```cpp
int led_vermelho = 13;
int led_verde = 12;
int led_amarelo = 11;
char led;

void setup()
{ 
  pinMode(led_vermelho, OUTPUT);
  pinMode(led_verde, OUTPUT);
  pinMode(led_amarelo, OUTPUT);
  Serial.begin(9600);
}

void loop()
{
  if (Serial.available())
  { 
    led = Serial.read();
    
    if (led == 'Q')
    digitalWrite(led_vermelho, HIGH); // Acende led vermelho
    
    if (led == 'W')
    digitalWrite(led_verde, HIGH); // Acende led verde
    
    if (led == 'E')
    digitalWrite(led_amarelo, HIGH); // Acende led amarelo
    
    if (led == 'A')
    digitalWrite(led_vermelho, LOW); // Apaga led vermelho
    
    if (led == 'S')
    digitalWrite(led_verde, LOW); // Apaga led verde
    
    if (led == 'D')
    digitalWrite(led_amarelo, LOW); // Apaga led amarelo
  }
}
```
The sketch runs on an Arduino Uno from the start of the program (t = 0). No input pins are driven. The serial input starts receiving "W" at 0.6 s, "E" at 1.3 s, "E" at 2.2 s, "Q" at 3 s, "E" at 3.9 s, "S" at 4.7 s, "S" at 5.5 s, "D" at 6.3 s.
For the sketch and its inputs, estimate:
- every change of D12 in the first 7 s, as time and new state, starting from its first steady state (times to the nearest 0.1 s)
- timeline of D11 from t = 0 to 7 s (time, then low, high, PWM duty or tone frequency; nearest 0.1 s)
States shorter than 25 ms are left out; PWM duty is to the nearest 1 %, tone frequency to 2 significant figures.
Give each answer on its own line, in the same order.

0 s low; 0.6 s high; 4.7 s low
0 s low; 1.3 s high; 6.3 s low
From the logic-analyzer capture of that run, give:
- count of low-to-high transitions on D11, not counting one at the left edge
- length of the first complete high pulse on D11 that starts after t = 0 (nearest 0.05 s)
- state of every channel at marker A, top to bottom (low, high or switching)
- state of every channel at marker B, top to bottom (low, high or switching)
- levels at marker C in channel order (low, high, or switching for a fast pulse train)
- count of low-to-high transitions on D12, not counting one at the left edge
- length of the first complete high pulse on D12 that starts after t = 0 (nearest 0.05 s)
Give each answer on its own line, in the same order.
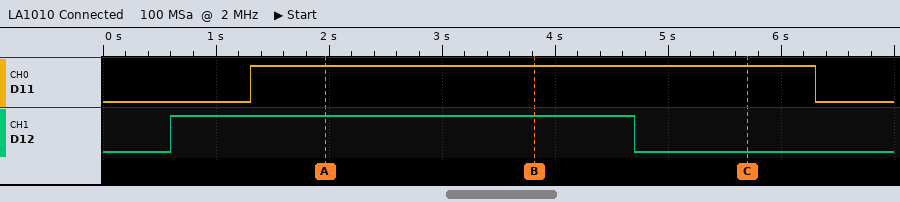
1
5.00 s
D11 high, D12 high
D11 high, D12 high
D11 high, D12 low
1
4.10 s
